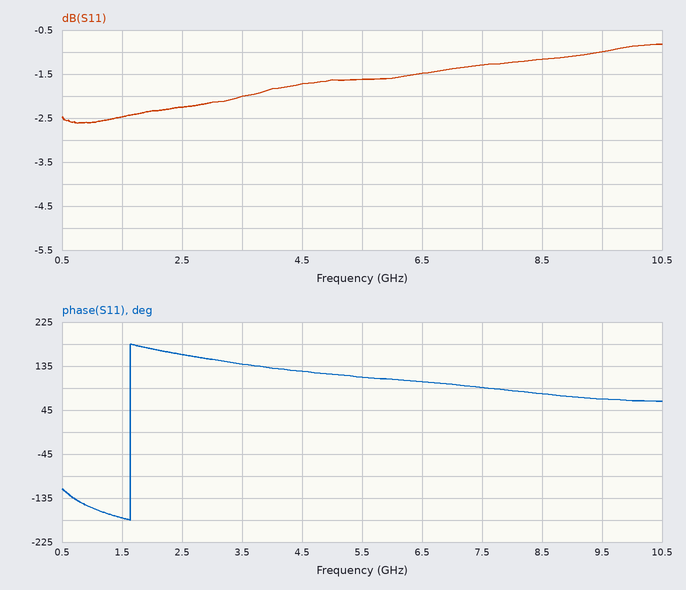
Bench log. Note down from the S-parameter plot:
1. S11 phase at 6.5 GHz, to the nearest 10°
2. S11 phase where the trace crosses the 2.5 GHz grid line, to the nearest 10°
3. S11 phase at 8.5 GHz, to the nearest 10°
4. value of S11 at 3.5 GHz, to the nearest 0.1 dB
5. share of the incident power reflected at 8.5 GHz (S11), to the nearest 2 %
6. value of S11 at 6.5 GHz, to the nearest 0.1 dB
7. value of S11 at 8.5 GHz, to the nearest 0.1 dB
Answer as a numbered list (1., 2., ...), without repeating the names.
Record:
1. 100°
2. 160°
3. 80°
4. -2.0 dB
5. 76 %
6. -1.5 dB
7. -1.2 dB
